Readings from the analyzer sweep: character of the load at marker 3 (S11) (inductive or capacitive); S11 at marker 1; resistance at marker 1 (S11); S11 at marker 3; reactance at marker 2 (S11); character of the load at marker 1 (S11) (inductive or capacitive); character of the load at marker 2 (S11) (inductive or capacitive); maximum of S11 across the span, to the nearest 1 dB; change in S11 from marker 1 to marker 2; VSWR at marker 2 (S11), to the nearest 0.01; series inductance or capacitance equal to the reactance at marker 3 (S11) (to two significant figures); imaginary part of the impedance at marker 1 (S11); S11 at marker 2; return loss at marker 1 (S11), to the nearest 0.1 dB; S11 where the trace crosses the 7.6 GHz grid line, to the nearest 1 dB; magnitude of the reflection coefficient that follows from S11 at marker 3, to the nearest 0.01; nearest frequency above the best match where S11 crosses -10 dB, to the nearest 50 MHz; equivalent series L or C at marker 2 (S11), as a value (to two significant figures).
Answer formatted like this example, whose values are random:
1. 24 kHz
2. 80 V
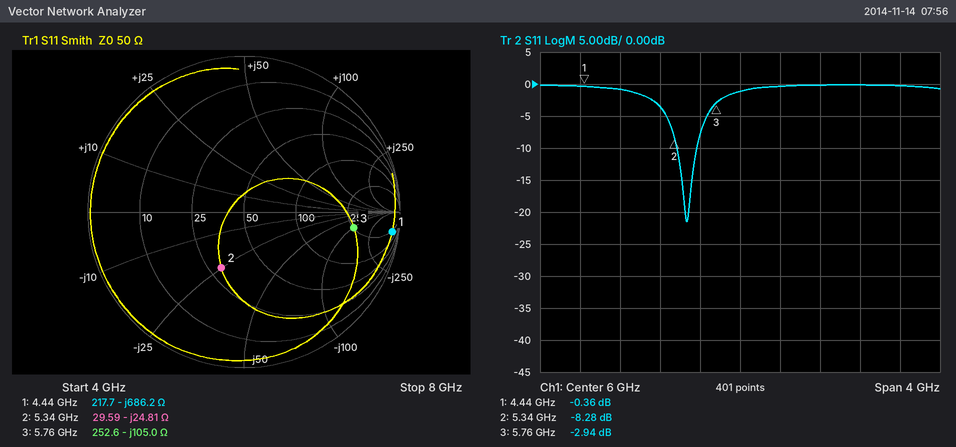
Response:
1. capacitive
2. -0.36 dB
3. 217.7 Ω
4. -2.94 dB
5. -24.81 Ω
6. capacitive
7. capacitive
8. 0 dB
9. -7.92 dB
10. 2.25
11. 260 fF
12. -686.2 Ω
13. -8.28 dB
14. 0.4 dB
15. 0 dB
16. 0.71
17. 5.55 GHz
18. 1.2 pF
